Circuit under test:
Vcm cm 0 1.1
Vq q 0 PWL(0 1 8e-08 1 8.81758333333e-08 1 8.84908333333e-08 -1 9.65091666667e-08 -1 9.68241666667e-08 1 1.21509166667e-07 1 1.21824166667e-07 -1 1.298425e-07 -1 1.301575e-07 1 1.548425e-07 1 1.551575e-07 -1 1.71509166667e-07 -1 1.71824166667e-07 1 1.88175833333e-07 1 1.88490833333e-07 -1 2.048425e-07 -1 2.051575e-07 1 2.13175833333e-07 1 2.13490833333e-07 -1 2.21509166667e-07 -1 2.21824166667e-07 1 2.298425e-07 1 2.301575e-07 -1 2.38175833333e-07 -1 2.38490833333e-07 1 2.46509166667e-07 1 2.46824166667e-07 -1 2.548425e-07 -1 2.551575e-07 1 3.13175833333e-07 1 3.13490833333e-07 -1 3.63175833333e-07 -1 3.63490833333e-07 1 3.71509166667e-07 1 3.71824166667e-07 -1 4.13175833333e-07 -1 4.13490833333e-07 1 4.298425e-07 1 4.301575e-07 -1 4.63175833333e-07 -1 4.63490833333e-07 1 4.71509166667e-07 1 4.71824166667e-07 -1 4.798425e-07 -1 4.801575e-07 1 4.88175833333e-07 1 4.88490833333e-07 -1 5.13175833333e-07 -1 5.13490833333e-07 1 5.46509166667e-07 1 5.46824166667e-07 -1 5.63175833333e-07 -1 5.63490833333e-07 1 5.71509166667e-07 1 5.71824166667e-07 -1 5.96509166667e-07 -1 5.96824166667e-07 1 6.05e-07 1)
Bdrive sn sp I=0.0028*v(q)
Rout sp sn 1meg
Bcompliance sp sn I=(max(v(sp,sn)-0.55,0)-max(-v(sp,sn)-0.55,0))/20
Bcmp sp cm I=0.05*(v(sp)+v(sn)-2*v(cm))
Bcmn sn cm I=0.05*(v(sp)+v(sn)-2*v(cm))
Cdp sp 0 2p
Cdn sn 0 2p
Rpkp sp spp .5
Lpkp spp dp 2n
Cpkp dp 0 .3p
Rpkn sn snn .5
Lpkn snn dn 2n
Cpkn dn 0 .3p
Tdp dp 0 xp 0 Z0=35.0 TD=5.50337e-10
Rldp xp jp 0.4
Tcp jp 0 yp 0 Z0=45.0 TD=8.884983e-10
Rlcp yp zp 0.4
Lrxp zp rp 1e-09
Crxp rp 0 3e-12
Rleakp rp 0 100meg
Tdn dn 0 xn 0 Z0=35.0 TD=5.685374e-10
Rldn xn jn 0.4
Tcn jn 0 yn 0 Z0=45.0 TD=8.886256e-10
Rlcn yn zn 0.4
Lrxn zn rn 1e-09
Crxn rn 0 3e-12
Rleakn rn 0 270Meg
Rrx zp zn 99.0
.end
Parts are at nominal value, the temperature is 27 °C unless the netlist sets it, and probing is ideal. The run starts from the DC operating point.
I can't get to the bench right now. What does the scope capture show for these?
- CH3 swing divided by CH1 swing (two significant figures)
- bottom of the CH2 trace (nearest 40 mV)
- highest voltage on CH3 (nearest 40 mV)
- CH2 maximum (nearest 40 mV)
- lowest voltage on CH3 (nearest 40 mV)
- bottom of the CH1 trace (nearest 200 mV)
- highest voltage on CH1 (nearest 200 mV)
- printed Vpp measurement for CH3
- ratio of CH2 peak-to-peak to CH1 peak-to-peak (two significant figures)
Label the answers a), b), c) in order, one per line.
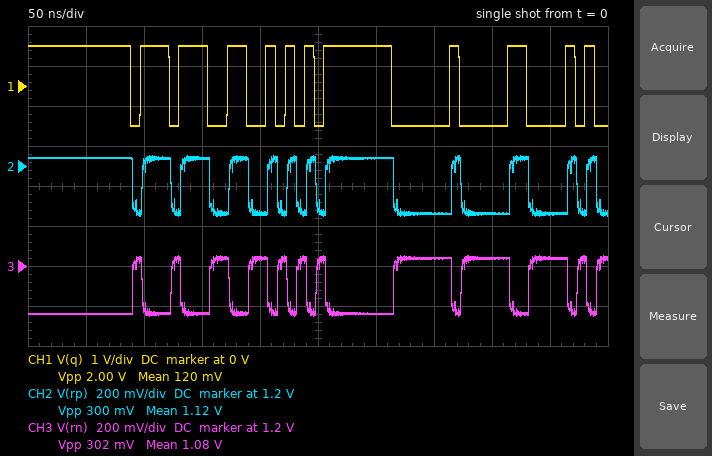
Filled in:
a) 0.15
b) 960 mV
c) 1.24 V
d) 1.24 V
e) 960 mV
f) -1.0 V
g) 1.0 V
h) 302 mV
i) 0.15
